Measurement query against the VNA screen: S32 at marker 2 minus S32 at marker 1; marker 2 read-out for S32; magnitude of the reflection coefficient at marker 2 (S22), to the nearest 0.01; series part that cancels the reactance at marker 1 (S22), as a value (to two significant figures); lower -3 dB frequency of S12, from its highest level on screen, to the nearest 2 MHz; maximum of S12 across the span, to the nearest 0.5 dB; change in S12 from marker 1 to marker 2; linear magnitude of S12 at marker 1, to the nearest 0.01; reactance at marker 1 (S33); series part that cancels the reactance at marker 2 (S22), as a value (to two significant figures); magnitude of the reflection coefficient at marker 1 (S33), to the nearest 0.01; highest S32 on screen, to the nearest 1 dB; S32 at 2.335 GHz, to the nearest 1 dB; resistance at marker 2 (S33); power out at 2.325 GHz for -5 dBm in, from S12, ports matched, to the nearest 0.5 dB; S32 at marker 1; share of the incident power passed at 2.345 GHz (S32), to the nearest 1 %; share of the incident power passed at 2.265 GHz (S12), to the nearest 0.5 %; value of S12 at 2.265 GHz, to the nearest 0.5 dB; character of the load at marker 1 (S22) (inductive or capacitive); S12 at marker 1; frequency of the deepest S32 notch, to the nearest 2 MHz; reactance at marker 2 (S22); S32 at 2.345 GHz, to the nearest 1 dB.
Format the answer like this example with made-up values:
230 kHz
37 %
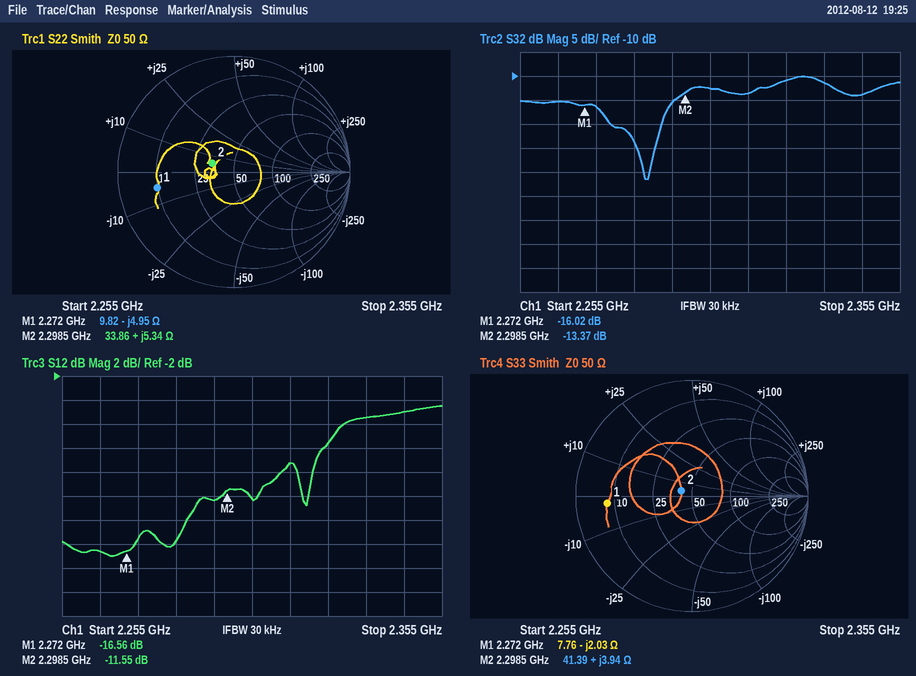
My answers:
2.65 dB
-13.37 dB
0.20
350 pH
2.326 GHz
-4.5 dB
5.01 dB
0.15
-2.03 Ω
13 pF
0.73
-10 dB
-11 dB
41.39 Ω
-12.5 dBm
-16.02 dB
4 %
2.0 %
-16.5 dB
capacitive
-16.56 dB
2.288 GHz
+5.34 Ω
-14 dB
